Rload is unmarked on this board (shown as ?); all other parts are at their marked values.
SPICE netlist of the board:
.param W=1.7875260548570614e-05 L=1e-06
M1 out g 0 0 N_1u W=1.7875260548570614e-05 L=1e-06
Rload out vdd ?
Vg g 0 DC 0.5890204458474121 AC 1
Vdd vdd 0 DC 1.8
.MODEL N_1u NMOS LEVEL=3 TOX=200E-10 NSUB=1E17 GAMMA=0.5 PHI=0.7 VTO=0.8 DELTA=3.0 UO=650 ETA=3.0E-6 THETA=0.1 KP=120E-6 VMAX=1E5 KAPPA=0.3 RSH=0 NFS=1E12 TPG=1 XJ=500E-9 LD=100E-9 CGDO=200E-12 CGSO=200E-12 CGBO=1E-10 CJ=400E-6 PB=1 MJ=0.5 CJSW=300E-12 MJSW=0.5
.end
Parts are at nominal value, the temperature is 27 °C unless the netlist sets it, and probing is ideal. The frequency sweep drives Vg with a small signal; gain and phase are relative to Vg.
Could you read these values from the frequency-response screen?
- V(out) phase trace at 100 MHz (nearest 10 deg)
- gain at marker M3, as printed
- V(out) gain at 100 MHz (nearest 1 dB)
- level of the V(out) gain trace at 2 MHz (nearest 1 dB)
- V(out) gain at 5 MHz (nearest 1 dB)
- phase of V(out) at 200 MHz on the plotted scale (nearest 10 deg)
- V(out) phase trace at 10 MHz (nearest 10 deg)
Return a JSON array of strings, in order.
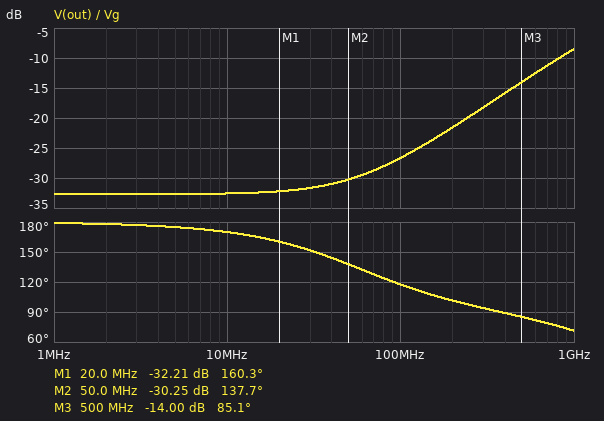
["120 deg", "-14.00 dB", "-27 dB", "-33 dB", "-33 dB", "100 deg", "170 deg"]
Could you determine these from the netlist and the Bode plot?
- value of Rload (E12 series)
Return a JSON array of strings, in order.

["18 kΩ"]
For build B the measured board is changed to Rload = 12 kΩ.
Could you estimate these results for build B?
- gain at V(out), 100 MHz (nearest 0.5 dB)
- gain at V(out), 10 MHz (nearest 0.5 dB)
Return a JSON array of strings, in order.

["-30.0 dB", "-36.0 dB"]
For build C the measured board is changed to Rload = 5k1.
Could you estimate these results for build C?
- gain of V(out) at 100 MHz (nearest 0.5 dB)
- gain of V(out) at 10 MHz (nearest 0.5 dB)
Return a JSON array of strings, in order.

["-37.5 dB", "-43.5 dB"]
